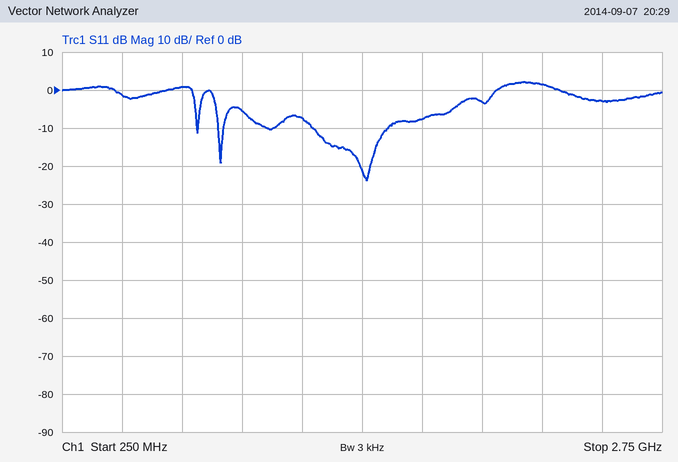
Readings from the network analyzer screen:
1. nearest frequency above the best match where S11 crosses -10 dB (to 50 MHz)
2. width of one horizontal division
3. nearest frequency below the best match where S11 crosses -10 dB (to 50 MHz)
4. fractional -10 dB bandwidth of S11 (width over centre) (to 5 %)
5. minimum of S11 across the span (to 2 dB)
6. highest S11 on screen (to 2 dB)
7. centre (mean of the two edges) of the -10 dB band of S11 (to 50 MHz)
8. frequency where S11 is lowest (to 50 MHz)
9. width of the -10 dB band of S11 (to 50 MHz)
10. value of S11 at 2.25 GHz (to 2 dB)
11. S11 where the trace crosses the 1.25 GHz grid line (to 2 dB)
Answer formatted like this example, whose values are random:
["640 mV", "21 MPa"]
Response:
["1.60 GHz", "250 MHz", "1.30 GHz", "20 %", "-24 dB", "2 dB", "1.45 GHz", "1.50 GHz", "300 MHz", "2 dB", "-8 dB"]
